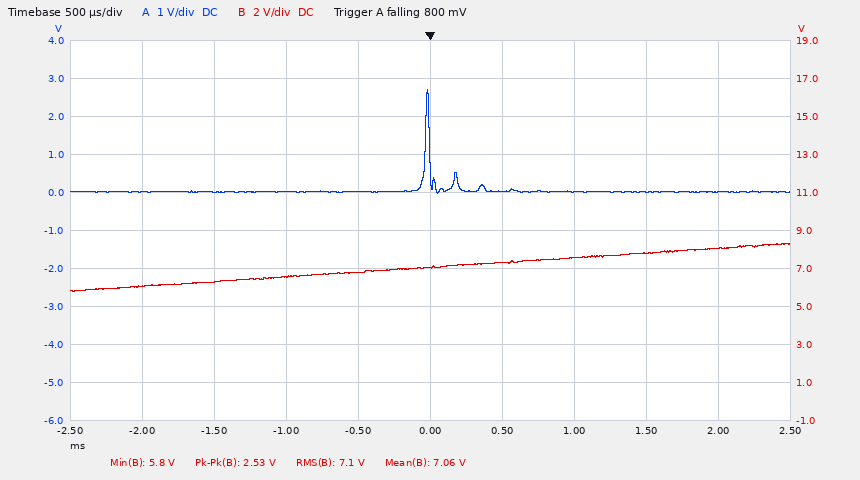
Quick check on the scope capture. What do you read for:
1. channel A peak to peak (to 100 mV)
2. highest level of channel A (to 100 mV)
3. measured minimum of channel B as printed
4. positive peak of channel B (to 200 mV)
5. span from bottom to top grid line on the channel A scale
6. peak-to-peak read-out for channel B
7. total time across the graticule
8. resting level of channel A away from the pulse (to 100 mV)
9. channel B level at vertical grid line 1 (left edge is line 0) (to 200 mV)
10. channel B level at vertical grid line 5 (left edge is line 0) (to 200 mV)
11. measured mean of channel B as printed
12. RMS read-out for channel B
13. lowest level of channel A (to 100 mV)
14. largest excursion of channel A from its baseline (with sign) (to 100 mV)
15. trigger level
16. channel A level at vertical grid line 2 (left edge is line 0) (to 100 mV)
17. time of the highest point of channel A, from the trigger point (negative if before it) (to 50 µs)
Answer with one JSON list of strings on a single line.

["2.7 V", "2.7 V", "5.8 V", "8.4 V", "10 V", "2.53 V", "5 ms", "0.0 V", "6.0 V", "7.0 V", "7.06 V", "7.1 V", "0.0 V", "+2.7 V", "800 mV", "0.0 V", "0 µs"]
